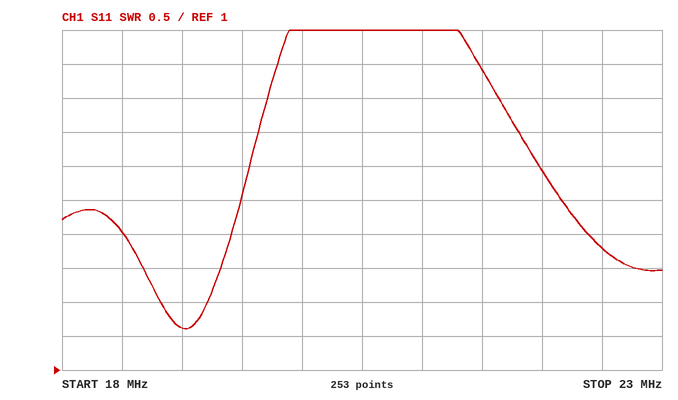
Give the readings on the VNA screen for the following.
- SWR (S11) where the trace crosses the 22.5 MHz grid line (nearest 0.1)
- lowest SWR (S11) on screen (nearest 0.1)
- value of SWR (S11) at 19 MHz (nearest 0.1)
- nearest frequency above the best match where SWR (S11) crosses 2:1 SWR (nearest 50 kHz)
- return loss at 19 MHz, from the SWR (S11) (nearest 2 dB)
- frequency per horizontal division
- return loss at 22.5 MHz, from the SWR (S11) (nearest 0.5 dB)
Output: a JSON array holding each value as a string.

["2.8", "1.6", "1.6", "19.20 MHz", "12 dB", "500 kHz", "6.5 dB"]
